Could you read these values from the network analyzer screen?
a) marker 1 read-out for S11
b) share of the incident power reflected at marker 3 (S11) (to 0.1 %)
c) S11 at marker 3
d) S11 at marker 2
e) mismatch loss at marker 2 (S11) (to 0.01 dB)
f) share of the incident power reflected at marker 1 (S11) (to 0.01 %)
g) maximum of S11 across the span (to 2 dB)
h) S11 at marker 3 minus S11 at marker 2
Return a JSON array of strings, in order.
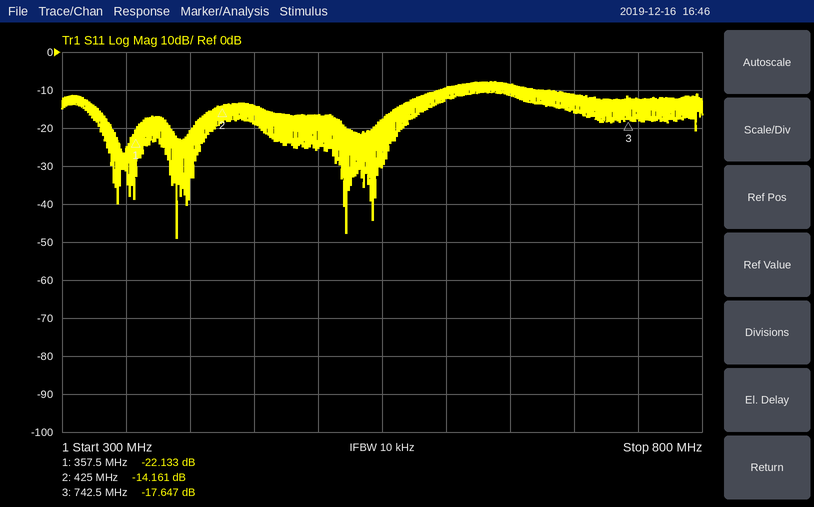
["-22.133 dB", "1.7 %", "-17.647 dB", "-14.161 dB", "0.17 dB", "0.61 %", "-8 dB", "-3.486 dB"]
